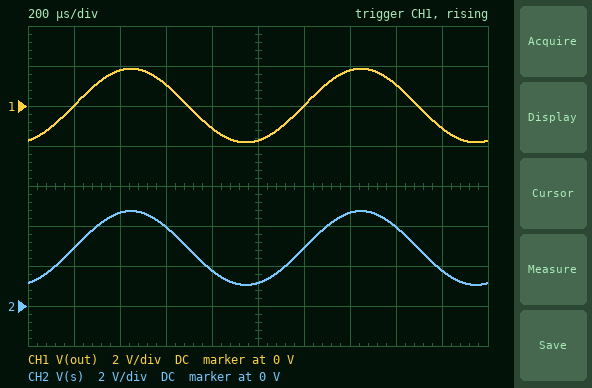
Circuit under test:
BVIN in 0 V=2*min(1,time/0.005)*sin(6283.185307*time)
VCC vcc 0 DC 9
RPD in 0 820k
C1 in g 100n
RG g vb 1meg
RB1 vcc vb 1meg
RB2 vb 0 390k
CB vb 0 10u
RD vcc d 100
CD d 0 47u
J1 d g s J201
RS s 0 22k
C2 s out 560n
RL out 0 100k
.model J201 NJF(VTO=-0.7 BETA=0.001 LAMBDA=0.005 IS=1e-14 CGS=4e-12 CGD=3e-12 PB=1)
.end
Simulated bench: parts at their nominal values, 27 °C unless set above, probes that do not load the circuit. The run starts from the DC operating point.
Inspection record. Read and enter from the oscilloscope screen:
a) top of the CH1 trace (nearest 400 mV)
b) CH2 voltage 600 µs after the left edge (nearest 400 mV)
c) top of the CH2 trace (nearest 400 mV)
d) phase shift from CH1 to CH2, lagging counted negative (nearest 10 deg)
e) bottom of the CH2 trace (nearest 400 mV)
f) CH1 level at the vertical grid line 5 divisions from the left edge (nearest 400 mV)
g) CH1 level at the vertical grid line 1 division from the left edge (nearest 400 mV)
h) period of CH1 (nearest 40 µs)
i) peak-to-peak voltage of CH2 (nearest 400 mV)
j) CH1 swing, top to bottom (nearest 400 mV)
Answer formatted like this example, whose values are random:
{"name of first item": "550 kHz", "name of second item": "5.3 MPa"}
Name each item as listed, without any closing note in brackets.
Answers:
{"top of the CH1 trace": "2.0 V", "CH2 voltage 600 µs after the left edge": "4.0 V", "top of the CH2 trace": "4.8 V", "phase shift from CH1 to CH2, lagging counted negative": "0 deg", "bottom of the CH2 trace": "1.2 V", "CH1 level at the vertical grid line 5 divisions from the left edge": "-1.6 V", "CH1 level at the vertical grid line 1 division from the left edge": "0 V", "period of CH1": "1.00 ms", "peak-to-peak voltage of CH2": "3.6 V", "CH1 swing, top to bottom": "3.6 V"}
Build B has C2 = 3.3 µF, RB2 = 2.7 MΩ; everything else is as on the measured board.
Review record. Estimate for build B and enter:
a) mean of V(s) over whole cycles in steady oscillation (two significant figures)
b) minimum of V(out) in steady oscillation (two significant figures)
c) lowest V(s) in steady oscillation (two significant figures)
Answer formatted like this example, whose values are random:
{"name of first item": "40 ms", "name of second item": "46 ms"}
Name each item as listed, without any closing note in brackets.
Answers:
{"mean of V(s) over whole cycles in steady oscillation": "6.7 V", "minimum of V(out) in steady oscillation": "-1.9 V", "lowest V(s) in steady oscillation": "4.8 V"}
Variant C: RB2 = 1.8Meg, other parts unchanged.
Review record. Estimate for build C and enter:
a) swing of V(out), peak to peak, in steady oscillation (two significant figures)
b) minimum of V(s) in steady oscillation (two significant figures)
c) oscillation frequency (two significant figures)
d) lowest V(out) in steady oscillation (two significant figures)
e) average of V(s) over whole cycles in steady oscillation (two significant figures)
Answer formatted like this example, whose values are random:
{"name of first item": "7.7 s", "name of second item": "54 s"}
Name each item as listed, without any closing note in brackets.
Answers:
{"swing of V(out), peak to peak, in steady oscillation": "3.8 V", "minimum of V(s) in steady oscillation": "4.1 V", "oscillation frequency": "1.0 kHz", "lowest V(out) in steady oscillation": "-1.9 V", "average of V(s) over whole cycles in steady oscillation": "6.0 V"}
